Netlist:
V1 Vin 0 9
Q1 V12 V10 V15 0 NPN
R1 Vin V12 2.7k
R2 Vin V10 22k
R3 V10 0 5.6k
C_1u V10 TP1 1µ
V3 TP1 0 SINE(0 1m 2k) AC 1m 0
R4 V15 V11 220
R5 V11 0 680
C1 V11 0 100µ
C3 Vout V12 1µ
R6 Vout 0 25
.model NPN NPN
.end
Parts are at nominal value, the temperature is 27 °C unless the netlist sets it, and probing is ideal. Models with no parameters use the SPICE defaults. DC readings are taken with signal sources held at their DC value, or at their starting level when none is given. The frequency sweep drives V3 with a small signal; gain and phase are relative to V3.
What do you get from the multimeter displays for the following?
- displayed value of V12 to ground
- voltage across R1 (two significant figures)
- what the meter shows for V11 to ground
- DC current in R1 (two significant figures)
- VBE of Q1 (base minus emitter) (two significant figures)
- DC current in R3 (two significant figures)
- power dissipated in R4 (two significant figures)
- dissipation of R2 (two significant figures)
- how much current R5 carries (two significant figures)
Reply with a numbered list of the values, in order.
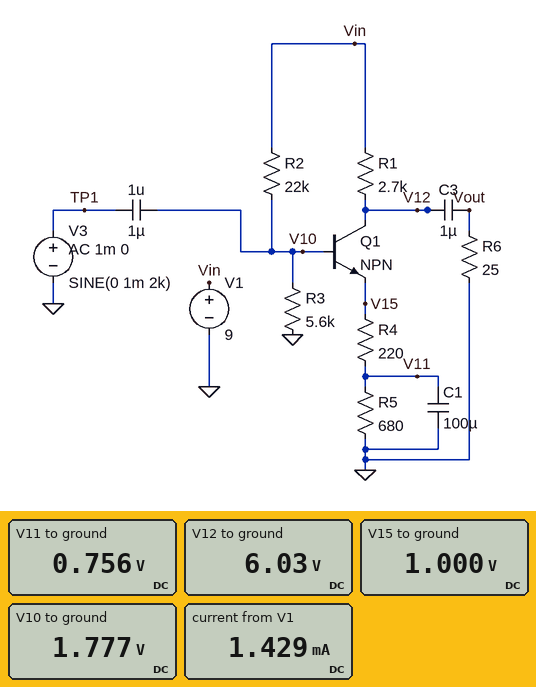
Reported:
1. 6.03 V
2. 3.0 V
3. 0.756 V
4. 1.1 mA
5. 780 mV
6. 320 µA
7. 270 µW
8. 2.4 mW
9. 1.1 mA
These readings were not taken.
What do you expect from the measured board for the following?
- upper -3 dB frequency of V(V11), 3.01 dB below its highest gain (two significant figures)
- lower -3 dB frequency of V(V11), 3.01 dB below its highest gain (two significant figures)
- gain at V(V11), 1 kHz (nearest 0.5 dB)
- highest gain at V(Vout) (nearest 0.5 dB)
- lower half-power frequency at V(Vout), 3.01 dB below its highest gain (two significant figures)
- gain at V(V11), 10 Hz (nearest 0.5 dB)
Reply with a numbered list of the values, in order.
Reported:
1. 57 Hz
2. 5.8 Hz
3. -43.5 dB
4. -20.0 dB
5. 80 Hz
6. -18.5 dB
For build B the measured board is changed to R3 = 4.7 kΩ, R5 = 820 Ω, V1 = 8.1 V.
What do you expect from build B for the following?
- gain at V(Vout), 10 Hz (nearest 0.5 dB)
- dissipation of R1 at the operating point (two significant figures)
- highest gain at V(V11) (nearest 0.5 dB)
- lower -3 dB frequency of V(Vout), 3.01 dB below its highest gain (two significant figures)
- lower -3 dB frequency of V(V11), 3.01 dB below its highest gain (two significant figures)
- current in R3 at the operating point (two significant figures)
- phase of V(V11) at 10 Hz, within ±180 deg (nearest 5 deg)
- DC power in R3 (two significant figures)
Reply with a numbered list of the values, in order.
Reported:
1. -51.5 dB
2. 1.0 mW
3. -19.0 dB
4. 83 Hz
5. 5.6 Hz
6. 300 µA
7. 25 deg
8. 420 µW
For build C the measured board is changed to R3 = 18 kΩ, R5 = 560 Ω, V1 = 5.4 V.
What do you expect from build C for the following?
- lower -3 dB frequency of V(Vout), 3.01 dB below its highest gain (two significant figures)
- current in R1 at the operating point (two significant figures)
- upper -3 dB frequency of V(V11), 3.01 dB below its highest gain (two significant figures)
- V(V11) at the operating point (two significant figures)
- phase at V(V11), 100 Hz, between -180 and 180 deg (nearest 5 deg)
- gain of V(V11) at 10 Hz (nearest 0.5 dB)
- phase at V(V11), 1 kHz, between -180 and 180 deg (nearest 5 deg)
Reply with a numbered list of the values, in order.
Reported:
1. 330 Hz
2. 1.5 mA
3. 570 Hz
4. 870 mV
5. 5 deg
6. -39.0 dB
7. -75 deg
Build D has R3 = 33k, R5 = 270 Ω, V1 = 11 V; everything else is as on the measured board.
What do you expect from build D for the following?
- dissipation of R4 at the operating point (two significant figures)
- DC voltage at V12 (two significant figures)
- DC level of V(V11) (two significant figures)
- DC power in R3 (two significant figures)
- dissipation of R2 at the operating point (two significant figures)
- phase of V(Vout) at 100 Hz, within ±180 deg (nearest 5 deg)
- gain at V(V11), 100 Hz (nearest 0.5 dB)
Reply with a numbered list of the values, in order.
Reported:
1. 3.0 mW
2. 1.9 V
3. 990 mV
4. 210 µW
5. 3.2 mW
6. 160 deg
7. -41.0 dB
